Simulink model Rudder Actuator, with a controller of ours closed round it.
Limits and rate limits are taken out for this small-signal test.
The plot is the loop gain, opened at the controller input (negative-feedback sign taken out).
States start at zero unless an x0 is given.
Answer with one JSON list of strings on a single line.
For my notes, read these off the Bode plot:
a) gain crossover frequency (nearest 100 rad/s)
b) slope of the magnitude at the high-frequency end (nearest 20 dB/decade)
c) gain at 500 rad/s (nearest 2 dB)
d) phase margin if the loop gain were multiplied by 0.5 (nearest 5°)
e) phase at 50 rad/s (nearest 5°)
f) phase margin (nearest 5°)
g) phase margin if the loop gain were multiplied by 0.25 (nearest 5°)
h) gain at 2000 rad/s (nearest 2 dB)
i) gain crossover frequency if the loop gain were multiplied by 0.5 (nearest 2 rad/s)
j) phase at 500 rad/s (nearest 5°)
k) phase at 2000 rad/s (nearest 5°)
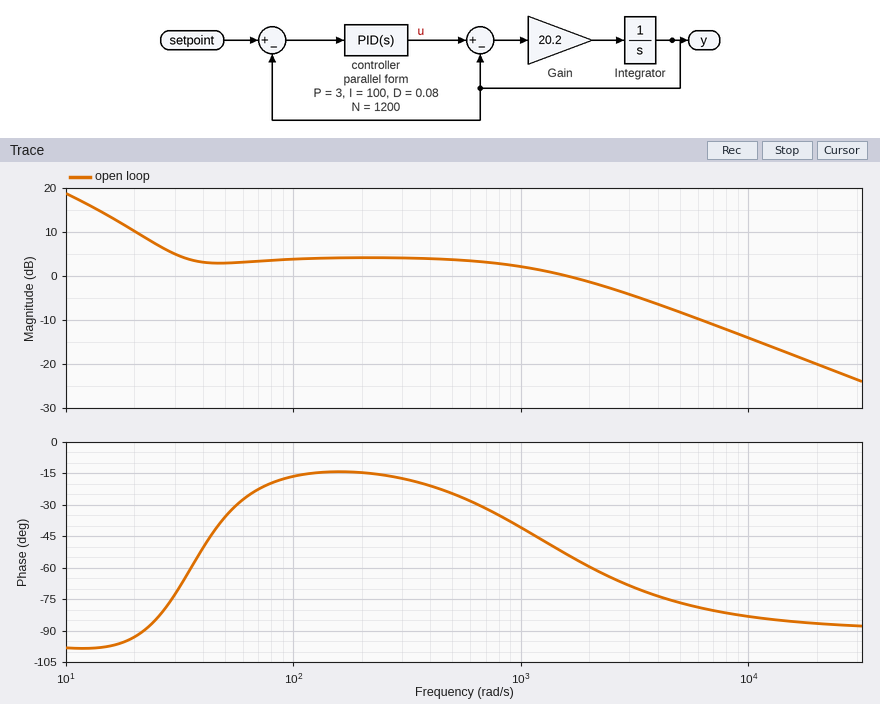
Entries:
["1600 rad/s", "-20 dB/decade", "4 dB", "100°", "-35°", "125°", "85°", "-2 dB", "28 rad/s", "-25°", "-60°"]
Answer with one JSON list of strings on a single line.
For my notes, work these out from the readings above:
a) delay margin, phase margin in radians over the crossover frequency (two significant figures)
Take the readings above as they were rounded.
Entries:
["0.0014 s"]
